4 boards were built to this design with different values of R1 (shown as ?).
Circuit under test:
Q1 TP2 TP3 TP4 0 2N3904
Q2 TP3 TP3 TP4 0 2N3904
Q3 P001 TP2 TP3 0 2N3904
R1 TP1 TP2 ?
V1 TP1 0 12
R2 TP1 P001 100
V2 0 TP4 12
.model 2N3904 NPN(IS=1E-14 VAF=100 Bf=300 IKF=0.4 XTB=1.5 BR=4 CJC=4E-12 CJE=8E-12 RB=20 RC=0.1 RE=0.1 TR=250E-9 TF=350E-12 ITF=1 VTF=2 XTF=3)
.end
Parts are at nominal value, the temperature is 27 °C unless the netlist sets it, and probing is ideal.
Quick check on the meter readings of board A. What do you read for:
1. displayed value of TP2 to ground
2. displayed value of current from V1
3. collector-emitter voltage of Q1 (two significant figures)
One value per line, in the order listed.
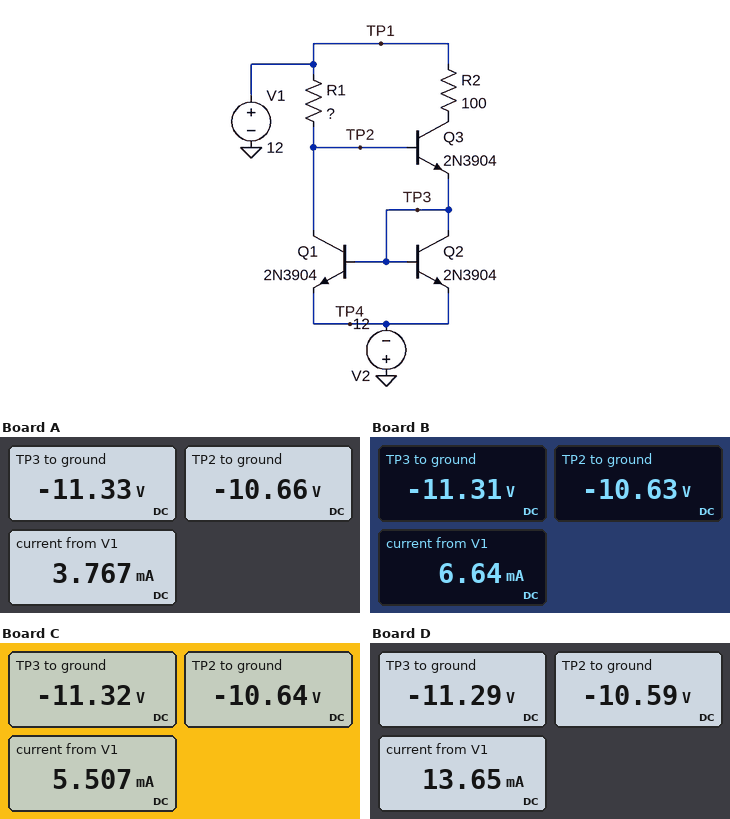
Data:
-10.66 V
3.767 mA
1.3 V
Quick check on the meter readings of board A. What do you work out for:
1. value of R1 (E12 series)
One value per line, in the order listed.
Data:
12 kΩ
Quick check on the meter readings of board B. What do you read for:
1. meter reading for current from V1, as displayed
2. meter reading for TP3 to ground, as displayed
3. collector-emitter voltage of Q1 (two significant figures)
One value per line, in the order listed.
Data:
6.64 mA
-11.31 V
1.4 V
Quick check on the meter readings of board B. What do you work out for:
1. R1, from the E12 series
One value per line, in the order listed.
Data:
6.8 kΩ
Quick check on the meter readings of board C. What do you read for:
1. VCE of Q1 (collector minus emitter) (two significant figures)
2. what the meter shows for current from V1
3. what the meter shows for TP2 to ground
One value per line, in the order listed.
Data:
1.4 V
5.507 mA
-10.64 V
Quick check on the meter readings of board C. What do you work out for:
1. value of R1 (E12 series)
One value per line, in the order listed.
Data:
8.2 kΩ
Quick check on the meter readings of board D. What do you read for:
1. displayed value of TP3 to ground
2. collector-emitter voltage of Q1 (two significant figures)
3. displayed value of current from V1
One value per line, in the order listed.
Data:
-11.29 V
1.4 V
13.65 mA
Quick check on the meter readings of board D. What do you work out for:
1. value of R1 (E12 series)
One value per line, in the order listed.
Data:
3.3 kΩ
